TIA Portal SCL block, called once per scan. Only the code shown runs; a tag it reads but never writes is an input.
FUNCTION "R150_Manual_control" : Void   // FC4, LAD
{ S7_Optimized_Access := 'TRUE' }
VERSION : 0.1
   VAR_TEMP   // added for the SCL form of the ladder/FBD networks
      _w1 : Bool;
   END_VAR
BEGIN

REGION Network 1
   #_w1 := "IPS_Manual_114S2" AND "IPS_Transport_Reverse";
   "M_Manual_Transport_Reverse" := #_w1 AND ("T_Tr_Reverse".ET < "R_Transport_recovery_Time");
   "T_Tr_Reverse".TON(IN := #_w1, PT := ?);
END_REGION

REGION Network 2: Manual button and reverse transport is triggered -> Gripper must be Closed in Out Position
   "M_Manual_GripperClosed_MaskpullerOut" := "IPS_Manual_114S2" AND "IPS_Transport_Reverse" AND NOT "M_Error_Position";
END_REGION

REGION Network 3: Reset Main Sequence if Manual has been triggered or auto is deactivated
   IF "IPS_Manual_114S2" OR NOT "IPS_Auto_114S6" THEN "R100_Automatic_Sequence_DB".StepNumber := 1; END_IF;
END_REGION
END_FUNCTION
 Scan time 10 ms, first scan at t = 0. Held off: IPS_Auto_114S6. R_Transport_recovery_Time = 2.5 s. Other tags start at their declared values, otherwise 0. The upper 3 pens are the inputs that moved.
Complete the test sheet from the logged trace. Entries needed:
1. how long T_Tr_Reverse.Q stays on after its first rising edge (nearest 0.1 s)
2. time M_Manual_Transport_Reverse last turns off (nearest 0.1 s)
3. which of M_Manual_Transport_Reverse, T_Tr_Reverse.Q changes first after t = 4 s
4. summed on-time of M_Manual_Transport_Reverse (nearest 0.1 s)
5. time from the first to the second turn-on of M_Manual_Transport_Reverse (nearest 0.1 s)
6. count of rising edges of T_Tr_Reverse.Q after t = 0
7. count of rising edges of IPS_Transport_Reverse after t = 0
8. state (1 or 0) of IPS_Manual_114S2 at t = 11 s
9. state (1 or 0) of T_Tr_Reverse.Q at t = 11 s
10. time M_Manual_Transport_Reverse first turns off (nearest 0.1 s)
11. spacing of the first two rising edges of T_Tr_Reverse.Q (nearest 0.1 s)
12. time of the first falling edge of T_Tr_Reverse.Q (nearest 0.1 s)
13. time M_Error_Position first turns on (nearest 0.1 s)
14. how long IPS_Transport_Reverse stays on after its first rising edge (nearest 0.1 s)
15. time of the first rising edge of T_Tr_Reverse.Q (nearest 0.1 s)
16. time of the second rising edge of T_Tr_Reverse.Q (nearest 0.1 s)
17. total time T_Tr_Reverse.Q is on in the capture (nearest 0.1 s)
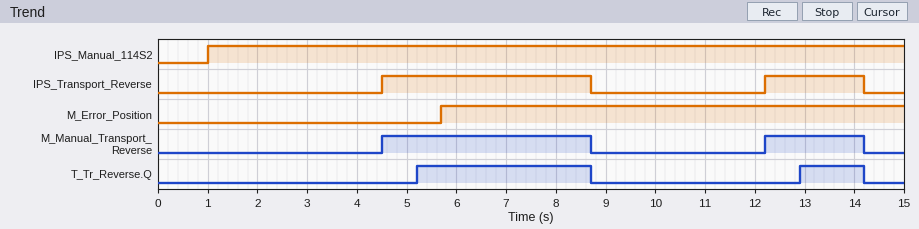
3.5 s
14.2 s
M_Manual_Transport_Reverse
6.2 s
7.7 s
2
2
1
0
8.7 s
7.7 s
8.7 s
5.7 s
4.2 s
5.2 s
12.9 s
4.8 s
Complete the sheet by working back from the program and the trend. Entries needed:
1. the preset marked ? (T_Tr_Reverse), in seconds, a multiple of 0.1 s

0.7 s
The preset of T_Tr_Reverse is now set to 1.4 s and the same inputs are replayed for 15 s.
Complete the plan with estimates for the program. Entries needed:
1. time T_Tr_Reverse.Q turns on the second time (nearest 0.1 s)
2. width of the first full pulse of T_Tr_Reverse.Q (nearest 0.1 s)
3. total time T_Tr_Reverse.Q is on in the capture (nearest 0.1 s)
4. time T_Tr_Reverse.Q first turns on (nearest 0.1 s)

13.6 s
2.8 s
3.4 s
5.9 s
